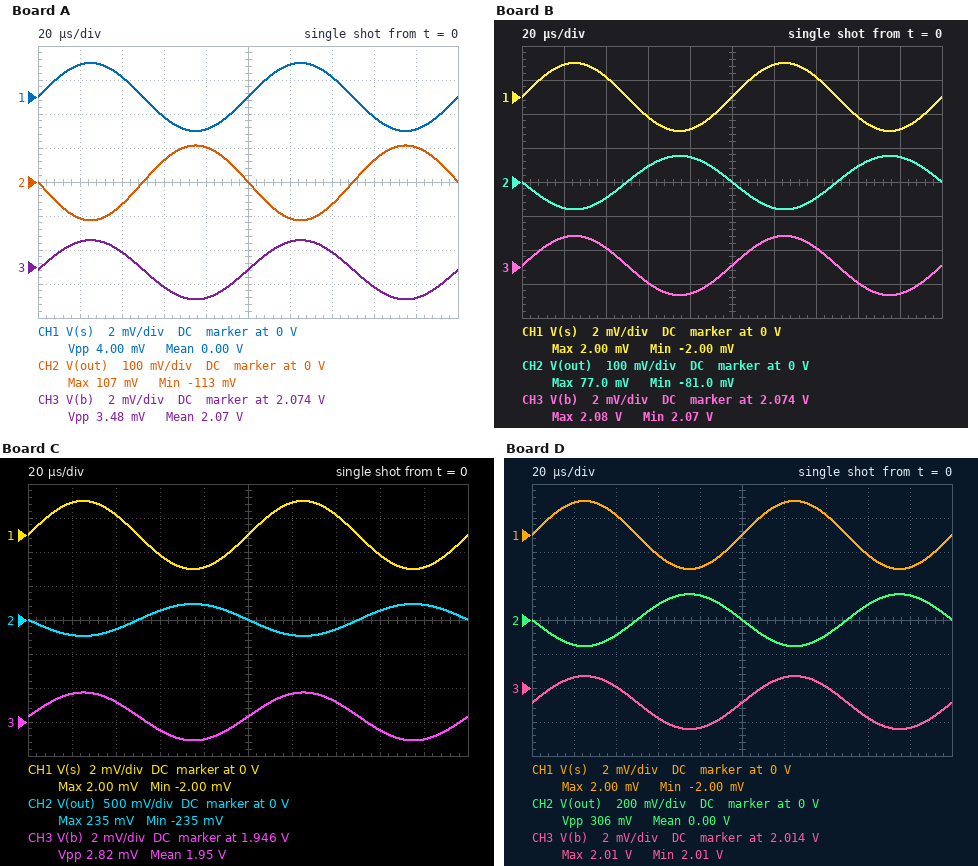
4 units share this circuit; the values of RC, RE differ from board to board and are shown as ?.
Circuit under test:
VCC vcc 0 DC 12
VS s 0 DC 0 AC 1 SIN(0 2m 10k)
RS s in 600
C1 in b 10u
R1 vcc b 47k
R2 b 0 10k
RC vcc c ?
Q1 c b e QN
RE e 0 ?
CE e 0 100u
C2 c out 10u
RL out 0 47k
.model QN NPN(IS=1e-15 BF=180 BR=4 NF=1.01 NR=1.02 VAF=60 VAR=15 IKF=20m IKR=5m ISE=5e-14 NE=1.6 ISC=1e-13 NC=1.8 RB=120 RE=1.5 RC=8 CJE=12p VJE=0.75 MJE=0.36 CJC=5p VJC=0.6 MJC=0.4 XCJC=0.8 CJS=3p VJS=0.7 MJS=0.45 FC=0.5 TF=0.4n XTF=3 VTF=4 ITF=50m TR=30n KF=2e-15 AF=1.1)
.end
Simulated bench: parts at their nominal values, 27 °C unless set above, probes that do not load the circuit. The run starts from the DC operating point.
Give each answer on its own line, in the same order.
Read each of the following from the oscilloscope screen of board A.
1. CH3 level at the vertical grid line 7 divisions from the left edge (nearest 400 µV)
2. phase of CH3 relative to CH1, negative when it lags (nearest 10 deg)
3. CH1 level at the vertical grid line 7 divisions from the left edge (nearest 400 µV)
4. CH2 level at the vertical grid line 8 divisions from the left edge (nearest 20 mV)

2.0748 V
0 deg
1.2 mV
60 mV
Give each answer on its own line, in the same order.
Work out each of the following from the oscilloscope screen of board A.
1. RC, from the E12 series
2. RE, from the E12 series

3.9 kΩ
2.7 kΩ
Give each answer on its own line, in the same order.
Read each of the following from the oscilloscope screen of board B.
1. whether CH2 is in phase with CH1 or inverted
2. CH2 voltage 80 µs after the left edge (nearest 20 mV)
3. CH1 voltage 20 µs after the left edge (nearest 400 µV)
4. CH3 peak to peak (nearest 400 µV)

inverted
80 mV
2.0 mV
3.6 mV
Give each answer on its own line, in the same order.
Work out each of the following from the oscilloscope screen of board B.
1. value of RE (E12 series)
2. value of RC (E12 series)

2.7 kΩ
2.7 kΩ
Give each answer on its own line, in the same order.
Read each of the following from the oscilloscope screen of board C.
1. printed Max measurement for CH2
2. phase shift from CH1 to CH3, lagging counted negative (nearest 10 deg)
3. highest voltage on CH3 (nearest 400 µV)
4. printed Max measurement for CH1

235 mV
0 deg
1.9476 V
2.00 mV
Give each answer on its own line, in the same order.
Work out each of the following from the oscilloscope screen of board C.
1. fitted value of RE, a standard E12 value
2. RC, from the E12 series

470 Ω
2.7 kΩ
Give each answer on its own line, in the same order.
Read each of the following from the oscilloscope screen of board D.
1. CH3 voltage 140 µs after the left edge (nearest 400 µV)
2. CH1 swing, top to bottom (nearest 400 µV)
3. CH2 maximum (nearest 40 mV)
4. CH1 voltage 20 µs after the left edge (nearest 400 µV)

2.0140 V
4.0 mV
160 mV
2.0 mV
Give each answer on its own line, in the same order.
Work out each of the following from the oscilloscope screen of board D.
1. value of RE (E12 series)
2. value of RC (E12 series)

820 Ω
2.2 kΩ
